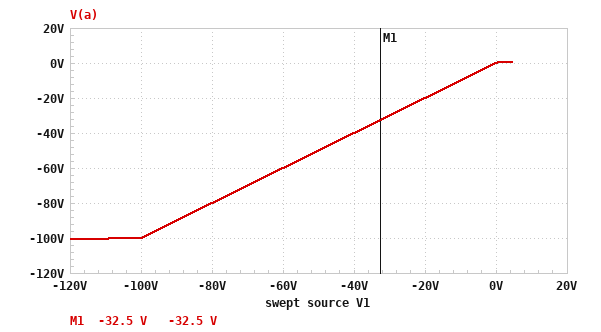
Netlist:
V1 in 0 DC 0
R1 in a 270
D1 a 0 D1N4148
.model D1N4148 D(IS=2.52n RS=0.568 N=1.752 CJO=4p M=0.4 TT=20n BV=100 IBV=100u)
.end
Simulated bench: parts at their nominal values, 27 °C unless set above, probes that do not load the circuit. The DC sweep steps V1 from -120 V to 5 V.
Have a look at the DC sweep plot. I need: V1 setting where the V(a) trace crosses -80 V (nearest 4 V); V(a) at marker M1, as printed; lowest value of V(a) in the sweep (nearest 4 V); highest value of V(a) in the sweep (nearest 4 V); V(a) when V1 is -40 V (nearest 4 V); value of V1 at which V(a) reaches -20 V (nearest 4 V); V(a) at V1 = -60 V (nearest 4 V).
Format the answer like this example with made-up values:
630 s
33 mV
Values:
-80 V
-32.5 V
-100 V
0 V
-40 V
-20 V
-60 V
